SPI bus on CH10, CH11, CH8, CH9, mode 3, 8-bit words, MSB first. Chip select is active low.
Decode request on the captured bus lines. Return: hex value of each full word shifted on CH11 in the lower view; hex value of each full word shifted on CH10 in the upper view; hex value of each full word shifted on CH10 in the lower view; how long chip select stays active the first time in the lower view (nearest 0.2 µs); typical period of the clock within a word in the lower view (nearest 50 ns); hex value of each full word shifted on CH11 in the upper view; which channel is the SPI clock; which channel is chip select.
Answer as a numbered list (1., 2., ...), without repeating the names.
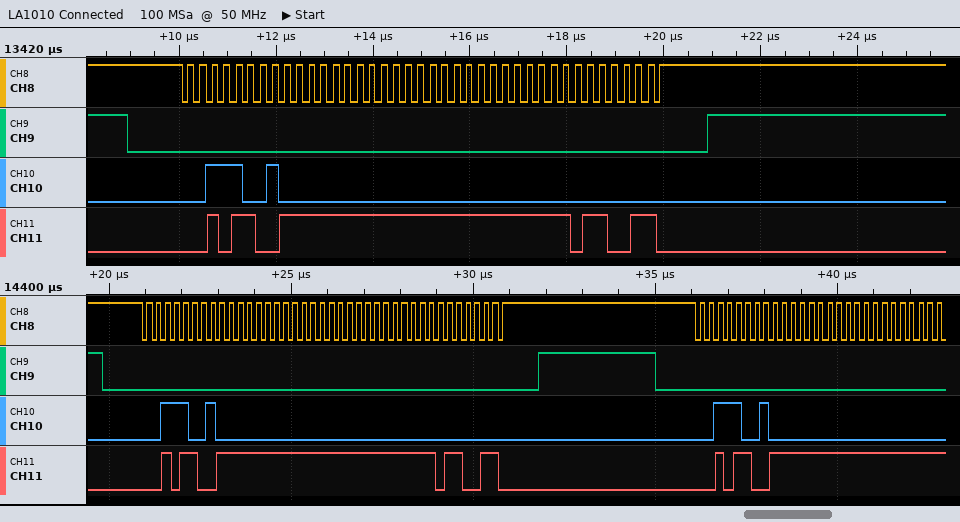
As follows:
1. 2C, FF, FF, FF, 66, 2C, FF, FF
2. 39, 00, 00, 00, 00
3. 39, 00, 00, 00, 00, 39, 00, 00
4. 12 µs
5. 250 ns
6. 2C, FF, FF, FF, 66
7. CH8
8. CH9
